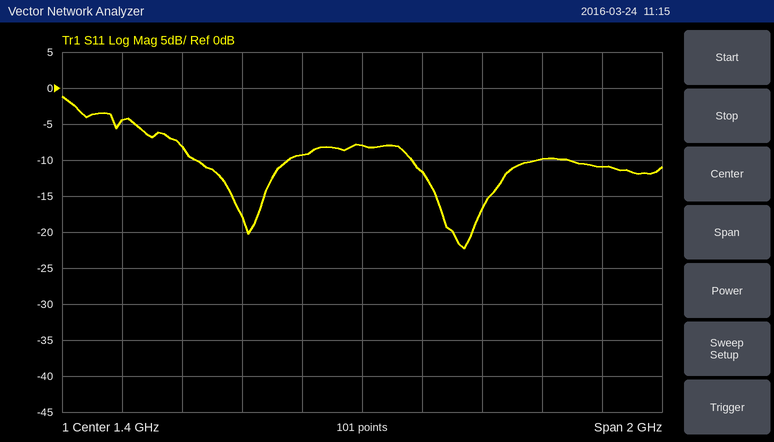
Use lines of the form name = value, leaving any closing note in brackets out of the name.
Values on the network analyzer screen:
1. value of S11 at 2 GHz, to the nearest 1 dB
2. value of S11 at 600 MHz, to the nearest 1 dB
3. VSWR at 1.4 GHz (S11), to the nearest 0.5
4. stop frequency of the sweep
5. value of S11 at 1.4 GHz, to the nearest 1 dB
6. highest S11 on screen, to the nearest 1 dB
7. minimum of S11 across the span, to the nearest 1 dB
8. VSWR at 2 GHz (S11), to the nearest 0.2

value of S11 at 2 GHz, to the nearest 1 dB = -10 dB
value of S11 at 600 MHz, to the nearest 1 dB = -4 dB
VSWR at 1.4 GHz (S11), to the nearest 0.5 = 2.5
stop frequency of the sweep = 2.4 GHz
value of S11 at 1.4 GHz, to the nearest 1 dB = -8 dB
highest S11 on screen, to the nearest 1 dB = -1 dB
minimum of S11 across the span, to the nearest 1 dB = -22 dB
VSWR at 2 GHz (S11), to the nearest 0.2 = 2.0
